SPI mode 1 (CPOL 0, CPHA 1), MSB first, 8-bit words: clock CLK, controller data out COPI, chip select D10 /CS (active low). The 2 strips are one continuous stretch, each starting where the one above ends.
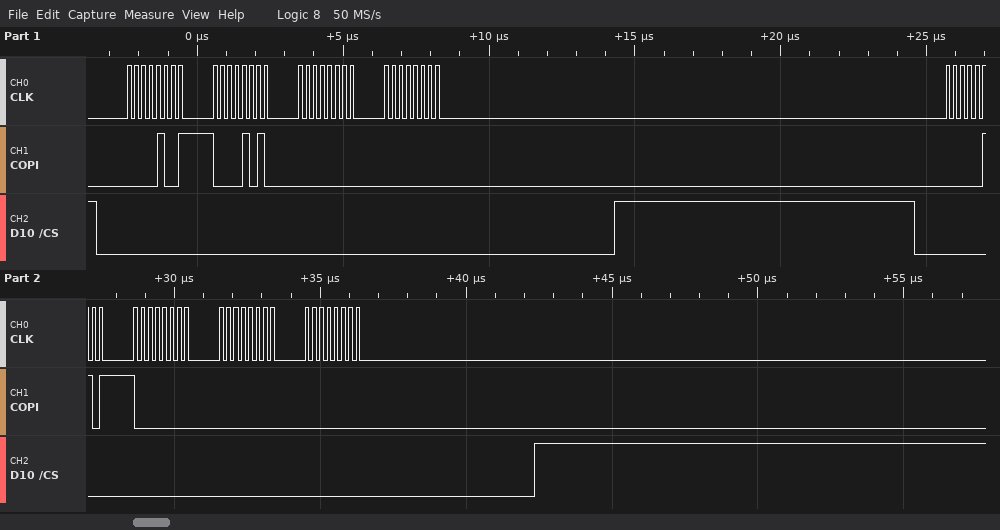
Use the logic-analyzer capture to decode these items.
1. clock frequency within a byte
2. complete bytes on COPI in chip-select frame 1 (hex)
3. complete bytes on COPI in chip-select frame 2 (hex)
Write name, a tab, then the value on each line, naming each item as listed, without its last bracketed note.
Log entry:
clock frequency within a byte	4 MHz
complete bytes on COPI in chip-select frame 1	09 0A 00 00
complete bytes on COPI in chip-select frame 2	05 00 00 00
